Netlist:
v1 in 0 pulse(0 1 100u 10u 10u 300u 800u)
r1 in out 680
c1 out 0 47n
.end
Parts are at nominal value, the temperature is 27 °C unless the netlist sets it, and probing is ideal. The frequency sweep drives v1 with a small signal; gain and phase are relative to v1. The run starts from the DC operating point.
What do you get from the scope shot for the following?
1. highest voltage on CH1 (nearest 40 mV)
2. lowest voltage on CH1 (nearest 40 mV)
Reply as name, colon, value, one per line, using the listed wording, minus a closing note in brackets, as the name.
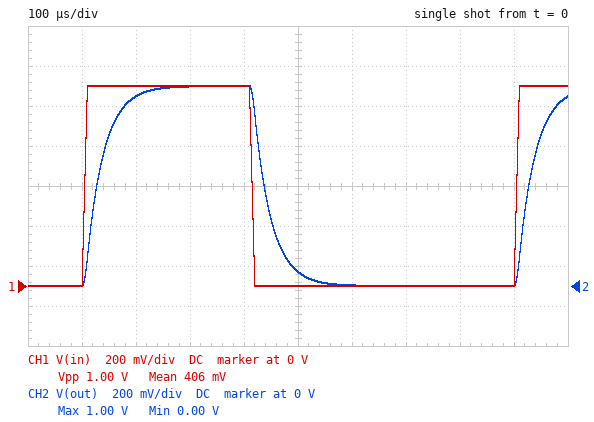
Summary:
highest voltage on CH1: 1.00 V
lowest voltage on CH1: 0 V
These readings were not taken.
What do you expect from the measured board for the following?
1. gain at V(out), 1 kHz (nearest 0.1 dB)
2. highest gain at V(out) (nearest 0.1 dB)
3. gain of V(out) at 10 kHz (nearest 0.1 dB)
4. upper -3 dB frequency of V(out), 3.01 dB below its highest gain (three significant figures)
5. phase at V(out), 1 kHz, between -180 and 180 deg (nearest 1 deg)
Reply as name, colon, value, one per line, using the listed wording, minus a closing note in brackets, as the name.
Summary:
gain at V(out), 1 kHz: -0.2 dB
highest gain at V(out): 0 dB
gain of V(out) at 10 kHz: -7.0 dB
upper -3 dB frequency of V(out), 3.01 dB below its highest gain: 4.98 kHz
phase at V(out), 1 kHz, between -180 and 180 deg: -11 deg
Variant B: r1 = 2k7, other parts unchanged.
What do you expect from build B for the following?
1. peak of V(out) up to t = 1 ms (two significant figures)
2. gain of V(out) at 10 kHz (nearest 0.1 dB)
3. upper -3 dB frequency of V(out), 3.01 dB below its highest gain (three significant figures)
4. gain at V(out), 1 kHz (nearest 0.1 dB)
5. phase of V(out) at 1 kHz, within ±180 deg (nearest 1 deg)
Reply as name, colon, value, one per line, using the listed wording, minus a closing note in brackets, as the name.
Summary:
peak of V(out) up to t = 1 ms: 910 mV
gain of V(out) at 10 kHz: -18.1 dB
upper -3 dB frequency of V(out), 3.01 dB below its highest gain: 1.25 kHz
gain at V(out), 1 kHz: -2.1 dB
phase of V(out) at 1 kHz, within ±180 deg: -39 deg
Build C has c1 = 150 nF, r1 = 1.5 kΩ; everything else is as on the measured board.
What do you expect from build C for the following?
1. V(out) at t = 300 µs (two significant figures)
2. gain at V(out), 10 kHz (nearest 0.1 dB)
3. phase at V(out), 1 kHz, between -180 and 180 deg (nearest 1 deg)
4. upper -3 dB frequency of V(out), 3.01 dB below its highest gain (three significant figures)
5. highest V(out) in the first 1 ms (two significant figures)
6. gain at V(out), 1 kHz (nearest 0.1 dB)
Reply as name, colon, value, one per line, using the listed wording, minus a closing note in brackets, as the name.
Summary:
V(out) at t = 300 µs: 580 mV
gain at V(out), 10 kHz: -23.0 dB
phase at V(out), 1 kHz, between -180 and 180 deg: -55 deg
upper -3 dB frequency of V(out), 3.01 dB below its highest gain: 707 Hz
highest V(out) in the first 1 ms: 740 mV
gain at V(out), 1 kHz: -4.8 dB
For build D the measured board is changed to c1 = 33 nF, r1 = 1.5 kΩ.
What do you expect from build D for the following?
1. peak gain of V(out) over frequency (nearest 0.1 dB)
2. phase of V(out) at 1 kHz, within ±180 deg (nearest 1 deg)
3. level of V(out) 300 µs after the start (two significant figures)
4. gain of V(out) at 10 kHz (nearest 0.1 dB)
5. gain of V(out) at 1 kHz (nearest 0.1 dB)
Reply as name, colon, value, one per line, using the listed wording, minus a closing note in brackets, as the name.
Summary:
peak gain of V(out) over frequency: 0 dB
phase of V(out) at 1 kHz, within ±180 deg: -17 deg
level of V(out) 300 µs after the start: 980 mV
gain of V(out) at 10 kHz: -10.3 dB
gain of V(out) at 1 kHz: -0.4 dB
